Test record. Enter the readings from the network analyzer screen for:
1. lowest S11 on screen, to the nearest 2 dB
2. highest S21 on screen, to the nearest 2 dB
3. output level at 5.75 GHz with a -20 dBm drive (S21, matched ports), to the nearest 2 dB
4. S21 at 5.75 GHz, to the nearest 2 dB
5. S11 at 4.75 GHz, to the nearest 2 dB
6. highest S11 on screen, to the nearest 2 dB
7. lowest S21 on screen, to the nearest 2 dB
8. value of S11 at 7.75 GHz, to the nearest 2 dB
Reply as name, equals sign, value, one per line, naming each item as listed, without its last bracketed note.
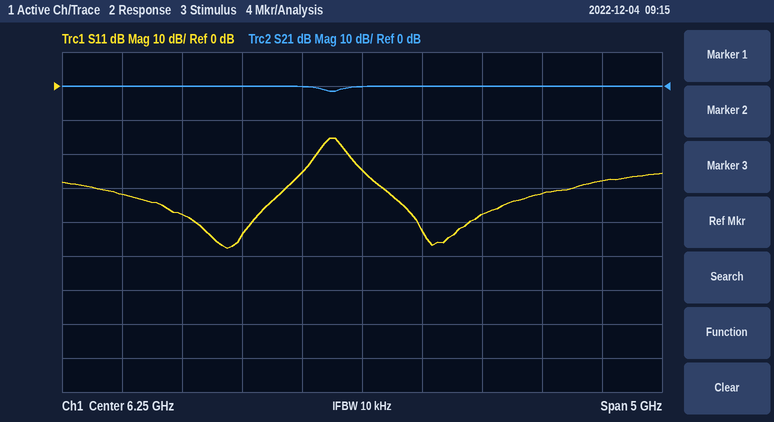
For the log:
lowest S11 on screen, to the nearest 2 dB = -48 dB
highest S21 on screen, to the nearest 2 dB = 0 dB
output level at 5.75 GHz with a -20 dBm drive (S21, matched ports), to the nearest 2 dB = -20 dBm
S21 at 5.75 GHz, to the nearest 2 dB = 0 dB
S11 at 4.75 GHz, to the nearest 2 dB = -38 dB
highest S11 on screen, to the nearest 2 dB = -16 dB
lowest S21 on screen, to the nearest 2 dB = -2 dB
value of S11 at 7.75 GHz, to the nearest 2 dB = -32 dB
